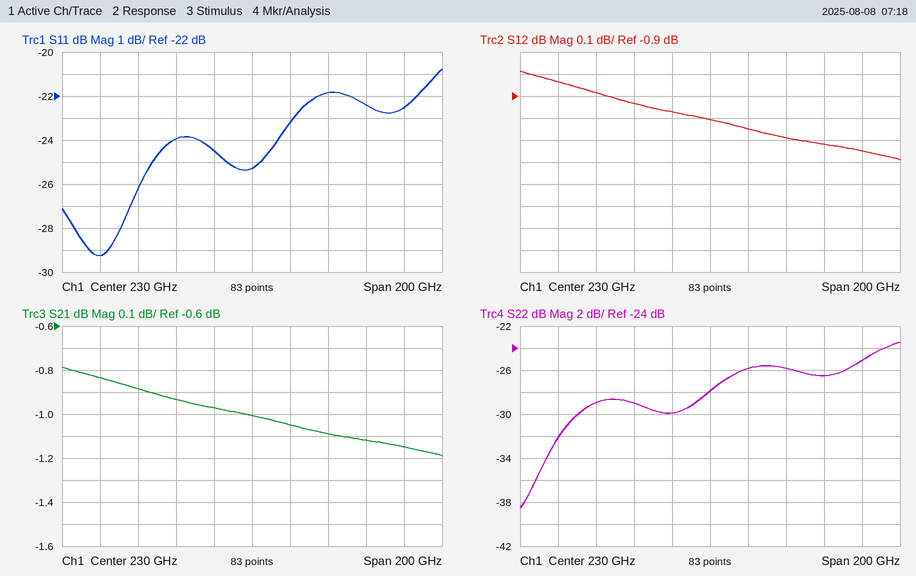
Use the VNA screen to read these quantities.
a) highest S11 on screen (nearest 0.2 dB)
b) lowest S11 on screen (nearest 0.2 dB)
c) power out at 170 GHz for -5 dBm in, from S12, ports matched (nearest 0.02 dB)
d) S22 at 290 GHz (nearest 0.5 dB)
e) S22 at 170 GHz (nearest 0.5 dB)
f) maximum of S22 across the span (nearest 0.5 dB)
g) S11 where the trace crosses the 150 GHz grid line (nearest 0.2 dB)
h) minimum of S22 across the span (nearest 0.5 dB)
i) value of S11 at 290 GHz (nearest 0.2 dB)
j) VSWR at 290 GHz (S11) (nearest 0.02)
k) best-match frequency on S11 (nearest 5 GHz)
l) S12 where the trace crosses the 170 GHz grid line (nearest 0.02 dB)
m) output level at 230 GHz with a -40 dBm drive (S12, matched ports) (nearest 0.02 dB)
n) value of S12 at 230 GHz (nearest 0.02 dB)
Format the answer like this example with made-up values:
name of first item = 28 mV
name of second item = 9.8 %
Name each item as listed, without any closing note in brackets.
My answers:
highest S11 on screen = -20.8 dB
lowest S11 on screen = -29.2 dB
power out at 170 GHz for -5 dBm in, from S12, ports matched = -5.88 dBm
S22 at 290 GHz = -26.5 dB
S22 at 170 GHz = -29.0 dB
maximum of S22 across the span = -23.5 dB
S11 where the trace crosses the 150 GHz grid line = -29.2 dB
minimum of S22 across the span = -38.5 dB
value of S11 at 290 GHz = -22.4 dB
VSWR at 290 GHz (S11) = 1.16
best-match frequency on S11 = 150 GHz
S12 where the trace crosses the 170 GHz grid line = -0.88 dB
output level at 230 GHz with a -40 dBm drive (S12, matched ports) = -41.00 dBm
value of S12 at 230 GHz = -1.00 dB
